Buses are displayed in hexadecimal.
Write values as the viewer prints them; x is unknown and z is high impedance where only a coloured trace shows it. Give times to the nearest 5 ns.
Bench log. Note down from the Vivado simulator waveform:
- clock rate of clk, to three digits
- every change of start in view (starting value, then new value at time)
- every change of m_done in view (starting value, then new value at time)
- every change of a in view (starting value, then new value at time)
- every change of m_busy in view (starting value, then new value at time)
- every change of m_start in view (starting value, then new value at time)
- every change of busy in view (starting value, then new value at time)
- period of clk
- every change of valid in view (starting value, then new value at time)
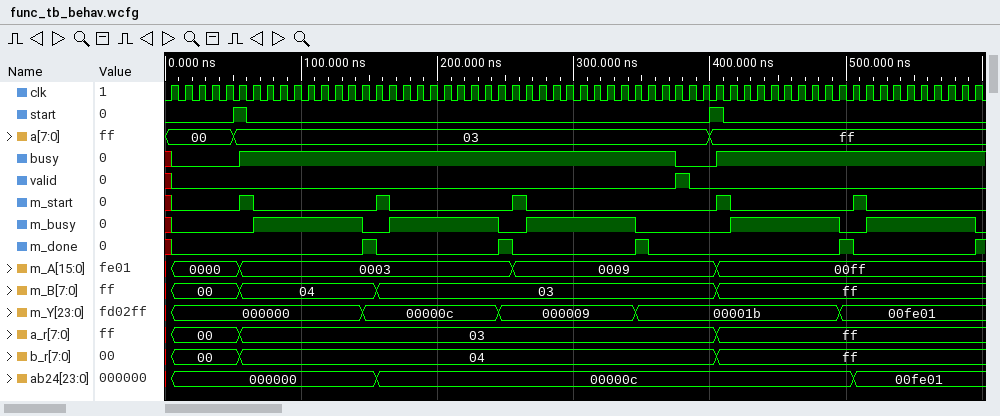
100 MHz
0, 1 at 50 ns, 0 at 60 ns, 1 at 400 ns, 0 at 410 ns
x, 0 at 5 ns, 1 at 145 ns, 0 at 155 ns, 1 at 245 ns, 0 at 255 ns, 1 at 345 ns, 0 at 355 ns, 1 at 495 ns, 0 at 505 ns, 1 at 595 ns
00, 03 at 50 ns, ff at 400 ns
x, 0 at 5 ns, 1 at 65 ns, 0 at 145 ns, 1 at 165 ns, 0 at 245 ns, 1 at 265 ns, 0 at 345 ns, 1 at 415 ns, 0 at 495 ns, 1 at 515 ns, 0 at 595 ns
x, 0 at 5 ns, 1 at 55 ns, 0 at 65 ns, 1 at 155 ns, 0 at 165 ns, 1 at 255 ns, 0 at 265 ns, 1 at 405 ns, 0 at 415 ns, 1 at 505 ns, 0 at 515 ns
x, 0 at 5 ns, 1 at 55 ns, 0 at 375 ns, 1 at 405 ns
10 ns
x, 0 at 5 ns, 1 at 375 ns, 0 at 385 ns
